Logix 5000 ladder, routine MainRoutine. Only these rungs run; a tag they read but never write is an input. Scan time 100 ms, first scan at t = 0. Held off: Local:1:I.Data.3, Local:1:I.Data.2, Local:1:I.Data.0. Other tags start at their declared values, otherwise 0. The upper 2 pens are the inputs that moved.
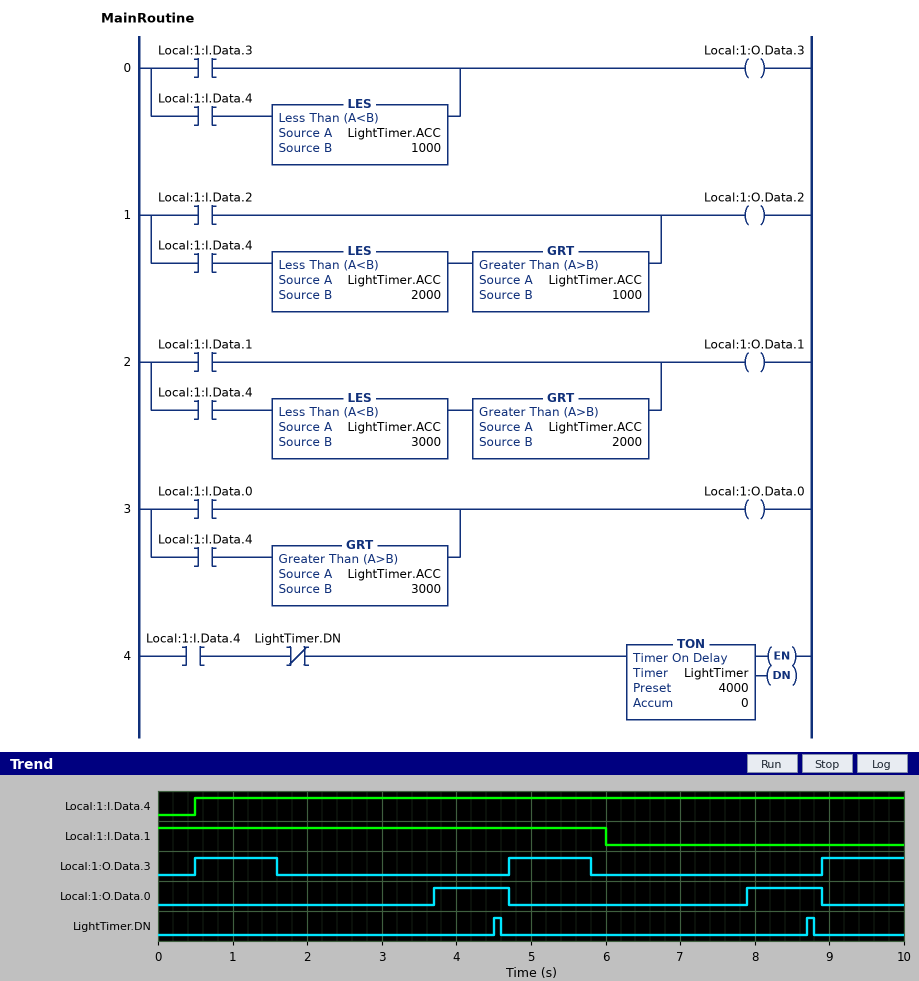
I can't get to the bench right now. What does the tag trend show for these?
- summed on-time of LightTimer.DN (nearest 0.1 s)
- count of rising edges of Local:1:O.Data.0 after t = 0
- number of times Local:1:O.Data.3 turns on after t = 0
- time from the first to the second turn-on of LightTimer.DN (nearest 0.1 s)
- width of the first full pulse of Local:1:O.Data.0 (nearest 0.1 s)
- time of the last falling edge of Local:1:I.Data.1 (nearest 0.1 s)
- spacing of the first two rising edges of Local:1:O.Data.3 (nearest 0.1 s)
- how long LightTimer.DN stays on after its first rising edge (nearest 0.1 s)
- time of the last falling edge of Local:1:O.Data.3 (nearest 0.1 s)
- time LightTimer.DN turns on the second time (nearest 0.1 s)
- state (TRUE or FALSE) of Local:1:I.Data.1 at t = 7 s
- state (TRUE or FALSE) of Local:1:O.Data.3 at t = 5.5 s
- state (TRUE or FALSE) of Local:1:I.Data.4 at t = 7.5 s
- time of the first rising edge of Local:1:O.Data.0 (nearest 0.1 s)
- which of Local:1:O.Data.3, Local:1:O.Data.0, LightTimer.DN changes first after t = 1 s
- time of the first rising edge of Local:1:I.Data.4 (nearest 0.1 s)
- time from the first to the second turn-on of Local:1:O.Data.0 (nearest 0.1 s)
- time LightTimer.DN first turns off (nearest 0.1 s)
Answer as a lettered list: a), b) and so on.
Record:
a) 0.2 s
b) 2
c) 3
d) 4.2 s
e) 1.0 s
f) 6.0 s
g) 4.2 s
h) 0.1 s
i) 5.8 s
j) 8.7 s
k) FALSE
l) TRUE
m) TRUE
n) 3.7 s
o) Local:1:O.Data.3
p) 0.5 s
q) 4.2 s
r) 4.6 s
